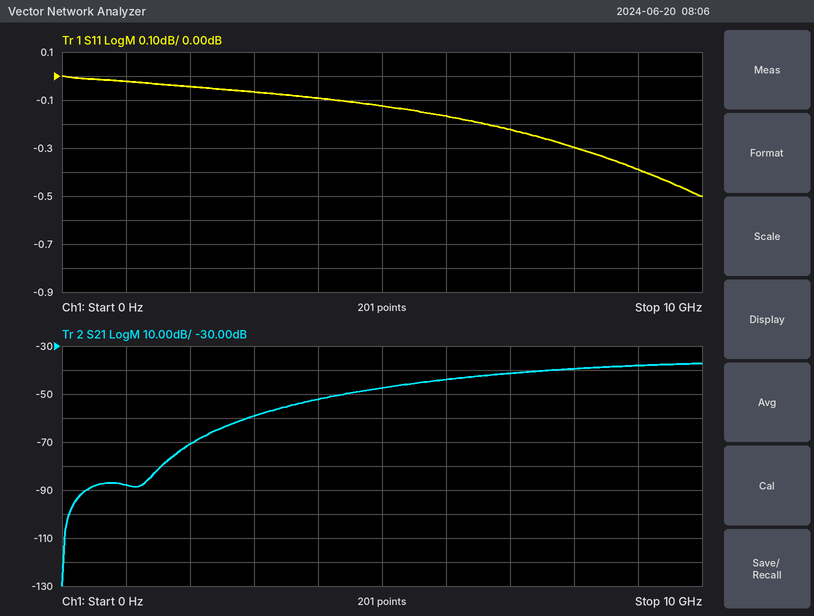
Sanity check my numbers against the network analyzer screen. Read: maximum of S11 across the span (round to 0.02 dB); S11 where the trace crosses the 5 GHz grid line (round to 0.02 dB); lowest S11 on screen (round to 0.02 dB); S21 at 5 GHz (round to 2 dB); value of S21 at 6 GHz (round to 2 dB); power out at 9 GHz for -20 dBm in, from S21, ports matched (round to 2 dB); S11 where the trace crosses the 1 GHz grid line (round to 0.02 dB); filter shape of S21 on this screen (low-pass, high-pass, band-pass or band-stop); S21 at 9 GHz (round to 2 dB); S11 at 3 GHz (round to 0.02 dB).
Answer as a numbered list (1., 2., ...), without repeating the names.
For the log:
1. 0.00 dB
2. -0.12 dB
3. -0.50 dB
4. -48 dB
5. -44 dB
6. -58 dBm
7. -0.02 dB
8. high-pass
9. -38 dB
10. -0.06 dB
